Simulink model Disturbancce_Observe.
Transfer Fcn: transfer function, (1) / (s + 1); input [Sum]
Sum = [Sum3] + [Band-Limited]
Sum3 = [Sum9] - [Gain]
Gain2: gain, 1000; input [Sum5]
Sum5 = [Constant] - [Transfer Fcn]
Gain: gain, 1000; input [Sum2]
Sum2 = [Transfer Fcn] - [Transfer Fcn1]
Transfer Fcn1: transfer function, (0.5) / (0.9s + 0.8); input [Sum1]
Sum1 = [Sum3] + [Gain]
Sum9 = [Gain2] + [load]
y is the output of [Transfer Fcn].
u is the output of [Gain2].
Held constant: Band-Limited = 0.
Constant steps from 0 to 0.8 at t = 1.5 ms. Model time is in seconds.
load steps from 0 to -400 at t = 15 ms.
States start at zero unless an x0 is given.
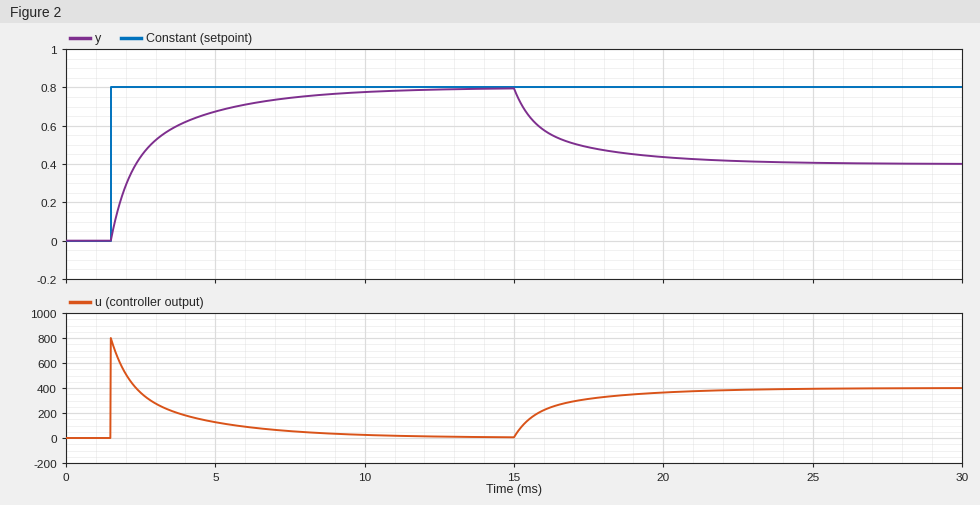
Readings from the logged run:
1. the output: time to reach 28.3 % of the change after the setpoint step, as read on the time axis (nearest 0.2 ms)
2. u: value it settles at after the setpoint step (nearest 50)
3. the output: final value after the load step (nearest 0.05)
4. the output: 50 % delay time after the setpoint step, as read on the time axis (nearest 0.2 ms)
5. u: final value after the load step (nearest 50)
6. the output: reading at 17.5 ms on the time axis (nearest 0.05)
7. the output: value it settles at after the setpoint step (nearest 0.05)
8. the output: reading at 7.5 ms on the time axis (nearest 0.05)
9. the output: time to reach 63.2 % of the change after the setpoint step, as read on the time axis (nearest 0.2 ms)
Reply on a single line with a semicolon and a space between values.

1.8 ms; 0; 0.40; 2.4 ms; 400; 0.50; 0.80; 0.75; 2.8 ms
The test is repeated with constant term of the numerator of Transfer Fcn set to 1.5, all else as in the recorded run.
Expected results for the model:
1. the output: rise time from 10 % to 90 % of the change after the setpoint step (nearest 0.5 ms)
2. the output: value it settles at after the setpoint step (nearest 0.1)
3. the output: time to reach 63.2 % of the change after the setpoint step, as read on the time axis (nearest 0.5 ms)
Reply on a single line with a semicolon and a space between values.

5.0 ms; 0.8; 2.5 ms
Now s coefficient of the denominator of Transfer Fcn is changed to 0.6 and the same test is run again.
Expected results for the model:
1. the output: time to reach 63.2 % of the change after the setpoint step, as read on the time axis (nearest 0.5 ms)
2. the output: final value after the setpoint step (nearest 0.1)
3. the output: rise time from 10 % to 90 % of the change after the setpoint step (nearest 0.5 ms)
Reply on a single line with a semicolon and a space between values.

2.5 ms; 0.8; 5.0 ms
